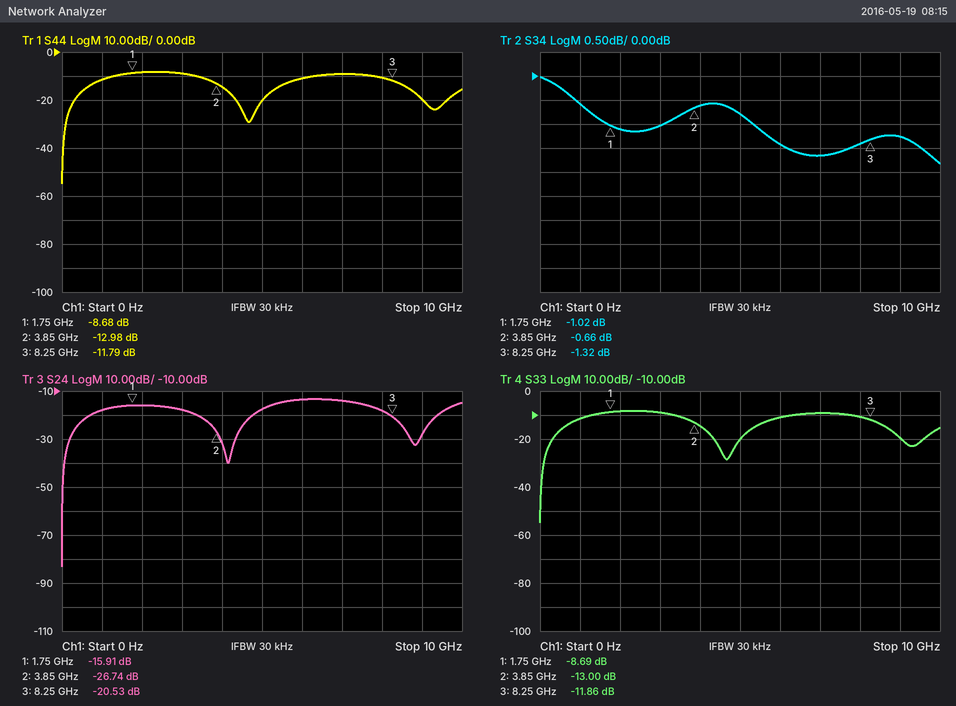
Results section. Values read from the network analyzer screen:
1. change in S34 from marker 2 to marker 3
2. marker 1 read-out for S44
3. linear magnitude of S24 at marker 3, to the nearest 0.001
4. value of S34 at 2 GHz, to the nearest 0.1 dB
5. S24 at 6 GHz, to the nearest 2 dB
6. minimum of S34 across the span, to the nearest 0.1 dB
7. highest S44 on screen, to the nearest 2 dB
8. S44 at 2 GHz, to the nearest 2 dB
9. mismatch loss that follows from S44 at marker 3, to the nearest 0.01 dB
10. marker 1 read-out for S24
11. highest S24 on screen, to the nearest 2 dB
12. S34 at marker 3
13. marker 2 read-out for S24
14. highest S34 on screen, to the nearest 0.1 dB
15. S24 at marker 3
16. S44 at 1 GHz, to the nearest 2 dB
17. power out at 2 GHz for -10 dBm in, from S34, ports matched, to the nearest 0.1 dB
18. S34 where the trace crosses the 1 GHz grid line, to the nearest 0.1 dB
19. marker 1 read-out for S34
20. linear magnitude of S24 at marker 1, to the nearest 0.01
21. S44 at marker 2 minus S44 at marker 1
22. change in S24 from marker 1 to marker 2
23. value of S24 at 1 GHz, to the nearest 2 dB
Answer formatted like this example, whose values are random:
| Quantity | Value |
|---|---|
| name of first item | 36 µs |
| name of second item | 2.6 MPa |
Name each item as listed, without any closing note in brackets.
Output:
| Quantity | Value |
|---|---|
| change in S34 from marker 2 to marker 3 | -0.66 dB |
| marker 1 read-out for S44 | -8.68 dB |
| linear magnitude of S24 at marker 3, to the nearest 0.001 | 0.094 |
| value of S34 at 2 GHz, to the nearest 0.1 dB | -1.1 dB |
| S24 at 6 GHz, to the nearest 2 dB | -14 dB |
| minimum of S34 across the span, to the nearest 0.1 dB | -1.8 dB |
| highest S44 on screen, to the nearest 2 dB | -8 dB |
| S44 at 2 GHz, to the nearest 2 dB | -8 dB |
| mismatch loss that follows from S44 at marker 3, to the nearest 0.01 dB | 0.30 dB |
| marker 1 read-out for S24 | -15.91 dB |
| highest S24 on screen, to the nearest 2 dB | -14 dB |
| S34 at marker 3 | -1.32 dB |
| marker 2 read-out for S24 | -26.74 dB |
| highest S34 on screen, to the nearest 0.1 dB | 0.0 dB |
| S24 at marker 3 | -20.53 dB |
| S44 at 1 GHz, to the nearest 2 dB | -12 dB |
| power out at 2 GHz for -10 dBm in, from S34, ports matched, to the nearest 0.1 dB | -11.1 dBm |
| S34 where the trace crosses the 1 GHz grid line, to the nearest 0.1 dB | -0.6 dB |
| marker 1 read-out for S34 | -1.02 dB |
| linear magnitude of S24 at marker 1, to the nearest 0.01 | 0.16 |
| S44 at marker 2 minus S44 at marker 1 | -4.30 dB |
| change in S24 from marker 1 to marker 2 | -10.83 dB |
| value of S24 at 1 GHz, to the nearest 2 dB | -18 dB |
